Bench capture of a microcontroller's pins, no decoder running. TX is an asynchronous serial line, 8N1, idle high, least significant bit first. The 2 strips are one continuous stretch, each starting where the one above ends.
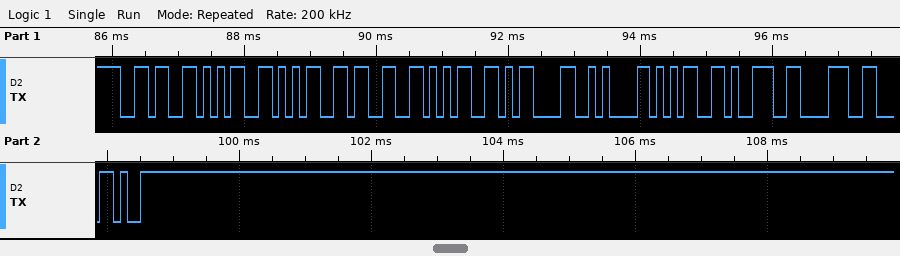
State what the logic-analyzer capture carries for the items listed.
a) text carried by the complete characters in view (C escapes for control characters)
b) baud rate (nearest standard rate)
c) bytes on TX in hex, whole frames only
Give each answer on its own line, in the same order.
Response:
"65535\r\n598,"
9600 baud
0x36 0x35 0x35 0x33 0x35 0x0D 0x0A 0x35 0x39 0x38 0x2C
